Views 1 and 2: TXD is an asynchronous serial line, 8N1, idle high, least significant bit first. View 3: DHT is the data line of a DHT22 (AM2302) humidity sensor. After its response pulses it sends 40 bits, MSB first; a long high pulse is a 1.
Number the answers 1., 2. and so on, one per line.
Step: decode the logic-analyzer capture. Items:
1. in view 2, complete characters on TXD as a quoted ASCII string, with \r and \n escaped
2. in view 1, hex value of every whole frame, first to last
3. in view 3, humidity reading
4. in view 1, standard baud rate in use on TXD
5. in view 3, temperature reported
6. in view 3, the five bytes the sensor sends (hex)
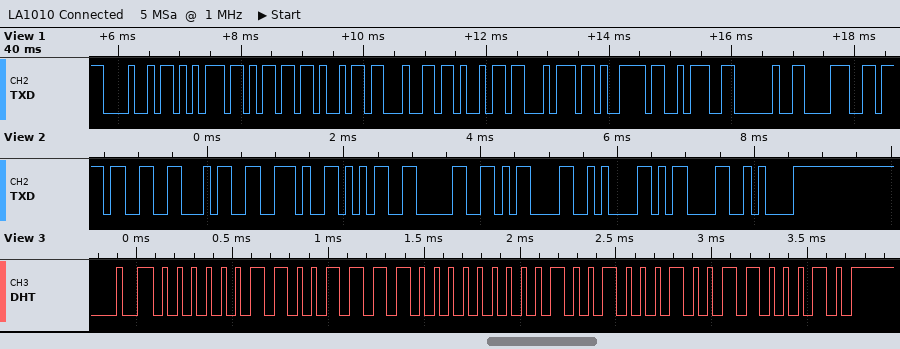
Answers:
1. "34.50\r\n\r\n"
2. 48 75 6D 69 64 69 74 79 3A 20 38
3. 82.8 %
4. 9600 baud
5. 29.0 °C
6. 03 3C 01 22 62
